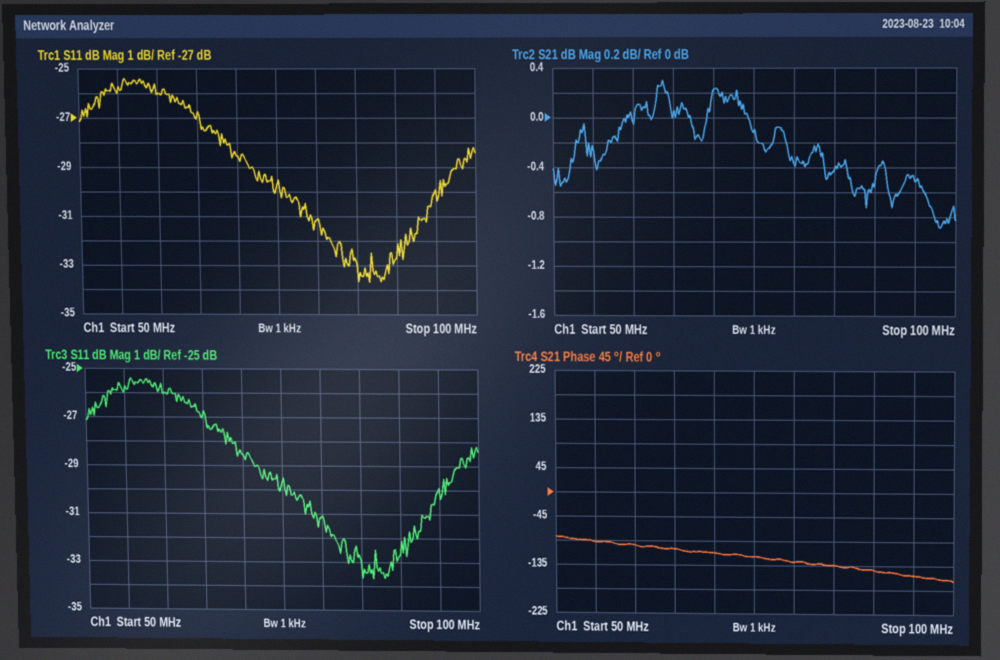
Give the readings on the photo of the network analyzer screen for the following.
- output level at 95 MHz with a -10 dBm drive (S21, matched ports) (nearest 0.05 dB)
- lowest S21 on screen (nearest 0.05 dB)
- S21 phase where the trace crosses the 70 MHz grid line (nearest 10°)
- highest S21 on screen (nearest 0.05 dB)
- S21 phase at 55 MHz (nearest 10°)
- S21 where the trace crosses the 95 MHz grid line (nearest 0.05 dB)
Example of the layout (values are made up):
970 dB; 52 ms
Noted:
-10.50 dBm; -0.90 dB; -110°; 0.30 dB; -90°; -0.50 dB
